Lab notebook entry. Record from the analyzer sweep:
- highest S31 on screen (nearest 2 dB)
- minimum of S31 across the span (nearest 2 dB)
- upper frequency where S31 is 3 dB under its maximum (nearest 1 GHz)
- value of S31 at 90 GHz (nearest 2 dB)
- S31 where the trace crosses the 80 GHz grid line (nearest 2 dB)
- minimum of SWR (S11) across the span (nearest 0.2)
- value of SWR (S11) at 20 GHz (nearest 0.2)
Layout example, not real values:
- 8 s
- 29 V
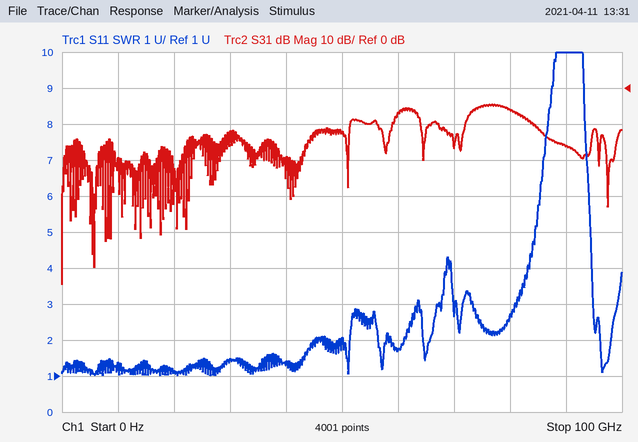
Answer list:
- -4 dB
- -54 dB
- 82 GHz
- -16 dB
- -6 dB
- 1.0
- 1.2
